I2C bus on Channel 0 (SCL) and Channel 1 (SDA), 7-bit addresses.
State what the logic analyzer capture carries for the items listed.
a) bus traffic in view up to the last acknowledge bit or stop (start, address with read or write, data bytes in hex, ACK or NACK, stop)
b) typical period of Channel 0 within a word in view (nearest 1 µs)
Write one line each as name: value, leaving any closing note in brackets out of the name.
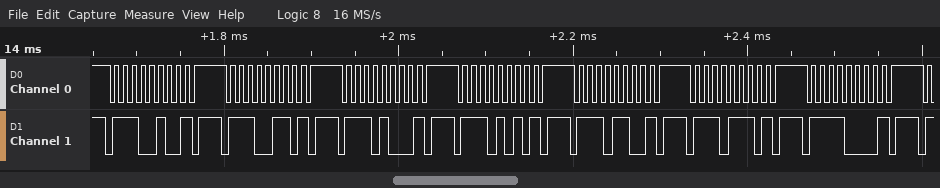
bus traffic in view up to the last acknowledge bit or stop: start, address 72 write NACK, stop, start, address 73 write NACK, stop, start, address 74 write NACK, stop, start, address 75 write NACK, stop, start, address 76 write NACK, stop, start, address 77 write NACK, stop, start, address 78 write NACK, stop
typical period of Channel 0 within a word in view: 10 µs
